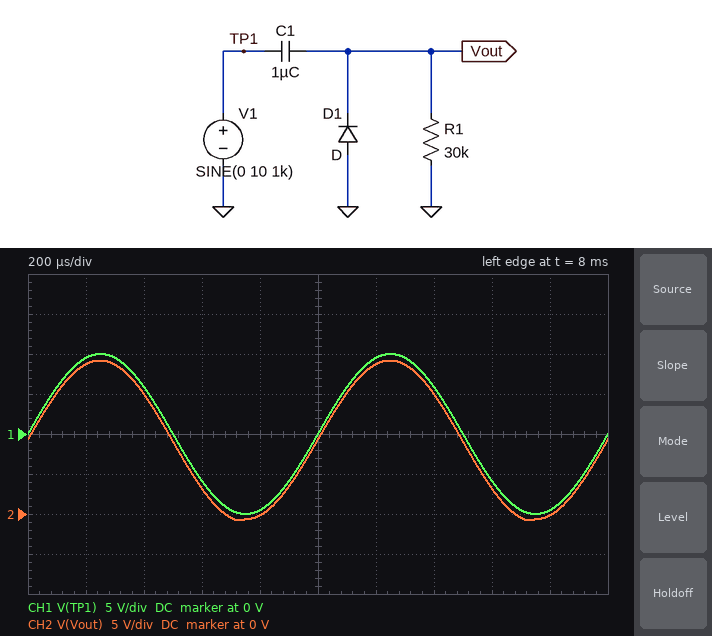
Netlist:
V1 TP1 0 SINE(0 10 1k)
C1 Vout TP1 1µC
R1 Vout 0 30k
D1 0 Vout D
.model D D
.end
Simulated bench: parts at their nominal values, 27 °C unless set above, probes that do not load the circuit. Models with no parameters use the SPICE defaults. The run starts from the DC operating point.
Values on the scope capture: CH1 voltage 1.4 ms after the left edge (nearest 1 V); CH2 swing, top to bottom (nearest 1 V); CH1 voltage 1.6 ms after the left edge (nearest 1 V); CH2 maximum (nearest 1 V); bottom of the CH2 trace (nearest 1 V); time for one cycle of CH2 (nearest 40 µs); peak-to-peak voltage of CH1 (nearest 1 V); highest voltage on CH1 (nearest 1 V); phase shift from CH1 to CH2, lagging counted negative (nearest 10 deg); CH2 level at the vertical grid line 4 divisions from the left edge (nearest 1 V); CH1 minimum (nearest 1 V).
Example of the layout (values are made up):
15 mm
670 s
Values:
6 V
20 V
-6 V
19 V
-1 V
1.00 ms
20 V
10 V
0 deg
0 V
-10 V
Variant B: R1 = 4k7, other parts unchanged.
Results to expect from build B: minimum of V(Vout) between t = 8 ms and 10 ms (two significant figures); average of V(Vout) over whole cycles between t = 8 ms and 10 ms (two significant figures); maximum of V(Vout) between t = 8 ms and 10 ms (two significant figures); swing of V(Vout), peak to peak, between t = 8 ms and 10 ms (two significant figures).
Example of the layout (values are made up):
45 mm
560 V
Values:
-750 mV
8.5 V
18 V
19 V
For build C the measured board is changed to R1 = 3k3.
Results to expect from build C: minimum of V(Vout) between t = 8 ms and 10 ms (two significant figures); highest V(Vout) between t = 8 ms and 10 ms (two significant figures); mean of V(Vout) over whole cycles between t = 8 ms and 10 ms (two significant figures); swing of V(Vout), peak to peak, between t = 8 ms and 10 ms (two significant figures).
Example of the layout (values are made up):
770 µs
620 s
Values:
-750 mV
18 V
8.2 V
19 V
